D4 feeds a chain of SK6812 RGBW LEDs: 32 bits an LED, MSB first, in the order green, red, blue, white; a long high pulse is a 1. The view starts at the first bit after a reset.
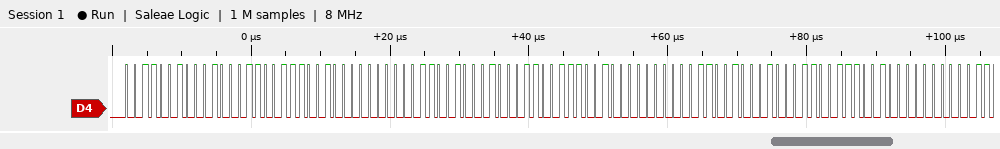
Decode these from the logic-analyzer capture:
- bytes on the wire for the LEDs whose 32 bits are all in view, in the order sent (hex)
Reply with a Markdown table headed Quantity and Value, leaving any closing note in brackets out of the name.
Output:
| Quantity | Value |
|---|---|
| bytes on the wire for the LEDs whose 32 bits are all in view, in the order sent | 32 23 39 00 32 23 39 00 32 23 39 00 |
